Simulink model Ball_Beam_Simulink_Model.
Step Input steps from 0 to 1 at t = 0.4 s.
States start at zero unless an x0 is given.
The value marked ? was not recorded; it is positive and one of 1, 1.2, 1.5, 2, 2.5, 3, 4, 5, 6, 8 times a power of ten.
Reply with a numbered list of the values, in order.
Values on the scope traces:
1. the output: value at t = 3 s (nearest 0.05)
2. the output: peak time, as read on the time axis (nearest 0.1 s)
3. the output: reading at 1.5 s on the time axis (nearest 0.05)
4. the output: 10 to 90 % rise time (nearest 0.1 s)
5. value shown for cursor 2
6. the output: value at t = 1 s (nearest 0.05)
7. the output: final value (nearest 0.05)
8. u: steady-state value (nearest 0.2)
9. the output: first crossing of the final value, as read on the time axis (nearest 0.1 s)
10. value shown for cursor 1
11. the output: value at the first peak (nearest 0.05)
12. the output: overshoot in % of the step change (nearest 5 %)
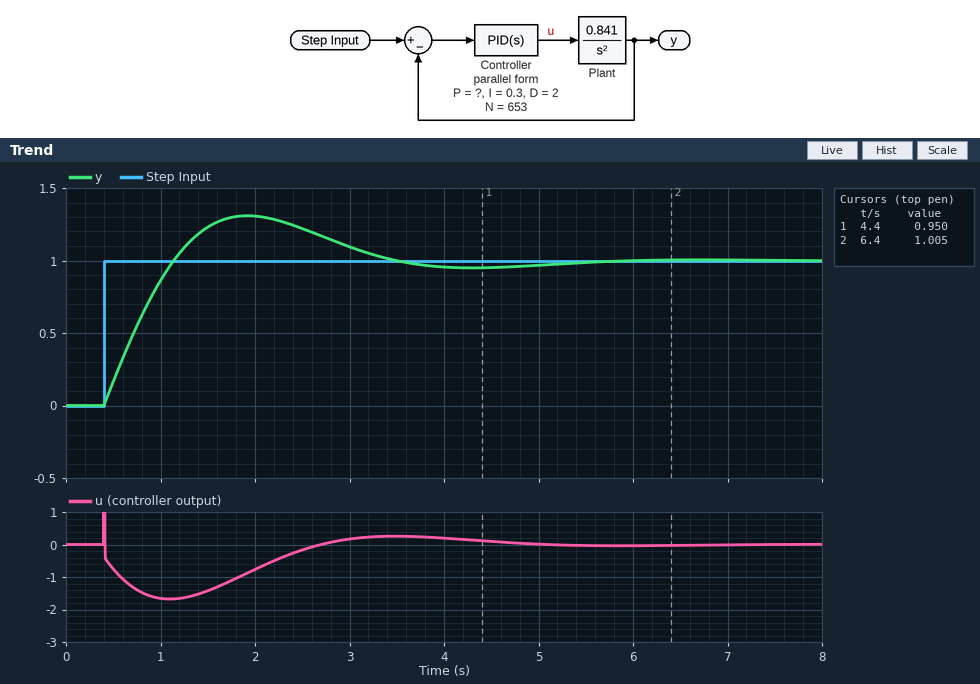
1. 1.10
2. 1.9 s
3. 1.25
4. 0.6 s
5. 1.005
6. 0.85
7. 1.00
8. 0.0
9. 1.1 s
10. 0.950
11. 1.30
12. 30 %
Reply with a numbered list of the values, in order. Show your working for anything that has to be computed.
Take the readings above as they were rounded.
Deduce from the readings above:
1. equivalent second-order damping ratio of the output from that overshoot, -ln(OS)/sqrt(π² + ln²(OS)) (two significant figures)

1. ln(0.3) = -1.204; 1.204 / sqrt(9.870 + 1.450) = 0.36
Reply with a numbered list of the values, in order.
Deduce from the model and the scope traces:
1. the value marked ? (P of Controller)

1. 3
